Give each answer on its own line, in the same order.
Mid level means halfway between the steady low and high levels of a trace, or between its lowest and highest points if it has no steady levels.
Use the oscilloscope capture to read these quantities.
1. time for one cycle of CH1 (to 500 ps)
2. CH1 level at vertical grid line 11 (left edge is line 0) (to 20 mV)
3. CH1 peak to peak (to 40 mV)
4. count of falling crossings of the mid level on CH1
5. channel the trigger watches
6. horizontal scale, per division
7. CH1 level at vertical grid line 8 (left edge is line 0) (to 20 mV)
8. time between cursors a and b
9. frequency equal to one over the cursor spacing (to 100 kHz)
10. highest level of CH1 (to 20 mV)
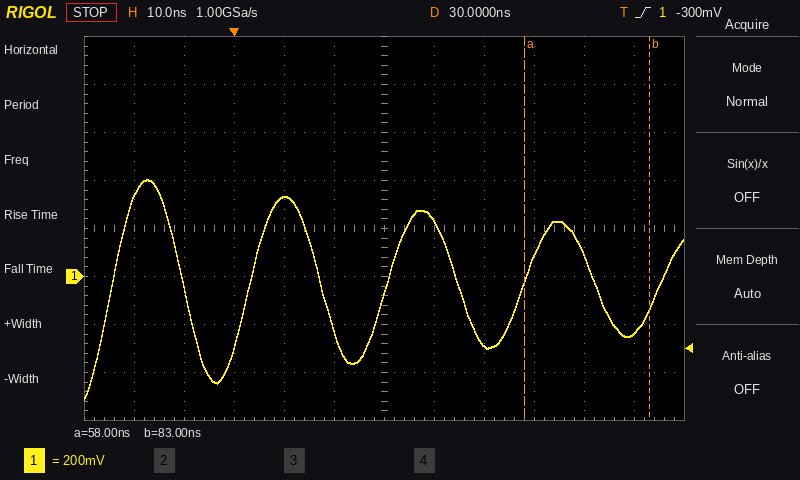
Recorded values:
27.5 ns
-240 mV
920 mV
4
CH1
10 ns
-280 mV
25 ns
40.0 MHz
400 mV
